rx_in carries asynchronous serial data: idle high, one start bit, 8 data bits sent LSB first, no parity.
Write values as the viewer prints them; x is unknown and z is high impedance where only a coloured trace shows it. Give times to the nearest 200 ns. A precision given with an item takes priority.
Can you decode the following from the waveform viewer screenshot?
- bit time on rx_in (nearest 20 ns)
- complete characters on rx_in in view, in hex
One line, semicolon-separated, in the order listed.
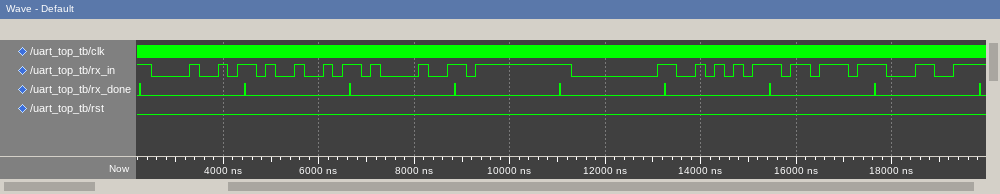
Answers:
200 ns; 48, 49, 21, FF, 00, AA, BB, CC
